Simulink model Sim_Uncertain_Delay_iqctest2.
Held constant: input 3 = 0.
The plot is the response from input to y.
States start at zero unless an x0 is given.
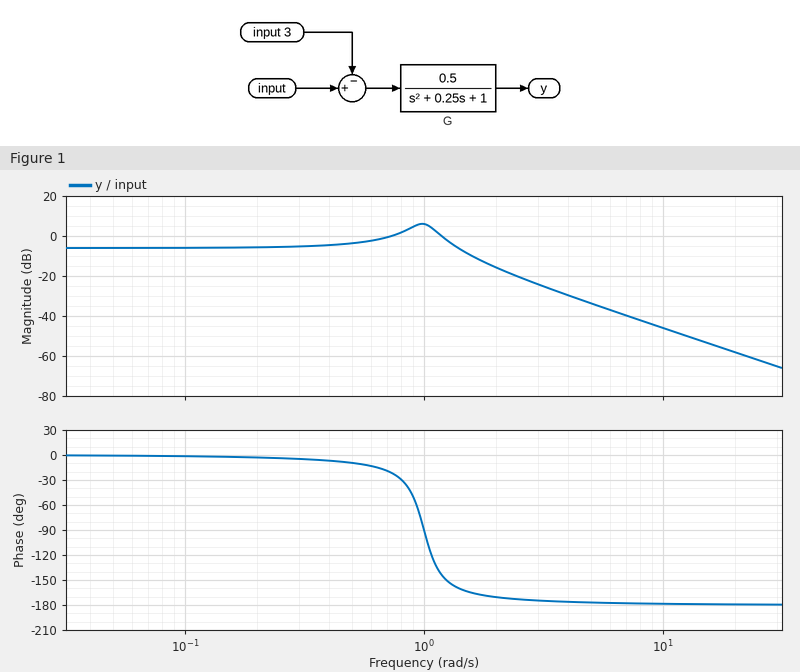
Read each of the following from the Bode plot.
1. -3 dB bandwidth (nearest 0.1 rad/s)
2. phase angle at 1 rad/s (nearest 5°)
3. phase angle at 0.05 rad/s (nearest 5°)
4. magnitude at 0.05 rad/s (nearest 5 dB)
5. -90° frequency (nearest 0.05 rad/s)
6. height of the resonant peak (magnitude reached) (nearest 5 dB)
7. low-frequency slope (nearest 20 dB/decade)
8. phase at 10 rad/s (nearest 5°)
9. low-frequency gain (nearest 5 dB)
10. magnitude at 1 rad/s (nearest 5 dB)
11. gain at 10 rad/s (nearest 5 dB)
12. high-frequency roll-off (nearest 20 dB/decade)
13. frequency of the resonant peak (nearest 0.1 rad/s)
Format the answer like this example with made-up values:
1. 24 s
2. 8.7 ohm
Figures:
1. 1.5 rad/s
2. -90°
3. 0°
4. -5 dB
5. 1.00 rad/s
6. 5 dB
7. 0 dB/decade
8. -180°
9. -5 dB
10. 5 dB
11. -45 dB
12. -40 dB/decade
13. 1.0 rad/s
